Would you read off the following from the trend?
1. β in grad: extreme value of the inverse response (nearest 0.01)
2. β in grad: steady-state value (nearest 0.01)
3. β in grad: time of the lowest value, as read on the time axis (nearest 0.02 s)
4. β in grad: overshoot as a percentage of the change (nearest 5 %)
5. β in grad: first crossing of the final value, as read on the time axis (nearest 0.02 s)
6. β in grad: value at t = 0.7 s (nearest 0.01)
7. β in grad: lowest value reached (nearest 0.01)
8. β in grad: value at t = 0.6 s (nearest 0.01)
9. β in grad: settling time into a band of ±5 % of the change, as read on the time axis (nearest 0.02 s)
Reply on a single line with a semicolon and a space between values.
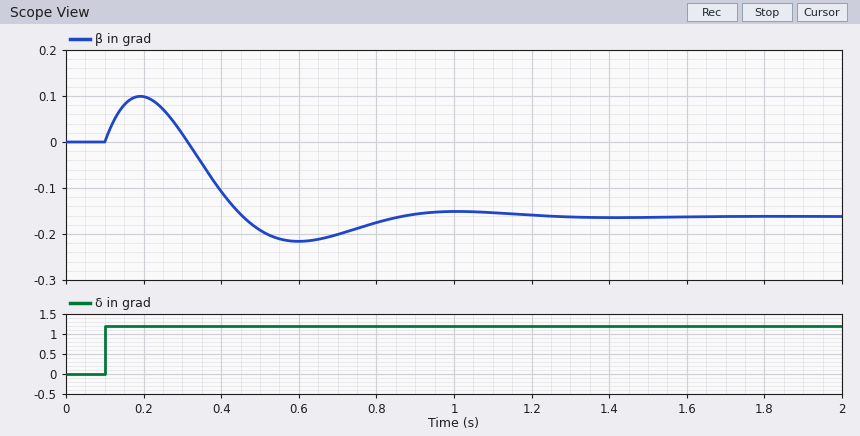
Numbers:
0.10; -0.16; 0.60 s; 35 %; 0.46 s; -0.20; -0.22; -0.22; 1.10 s
